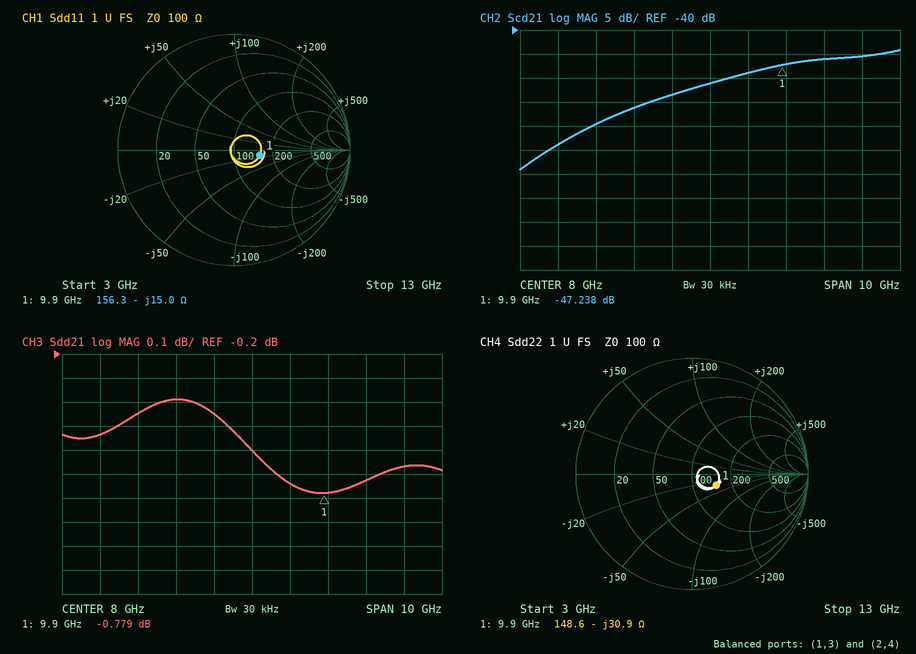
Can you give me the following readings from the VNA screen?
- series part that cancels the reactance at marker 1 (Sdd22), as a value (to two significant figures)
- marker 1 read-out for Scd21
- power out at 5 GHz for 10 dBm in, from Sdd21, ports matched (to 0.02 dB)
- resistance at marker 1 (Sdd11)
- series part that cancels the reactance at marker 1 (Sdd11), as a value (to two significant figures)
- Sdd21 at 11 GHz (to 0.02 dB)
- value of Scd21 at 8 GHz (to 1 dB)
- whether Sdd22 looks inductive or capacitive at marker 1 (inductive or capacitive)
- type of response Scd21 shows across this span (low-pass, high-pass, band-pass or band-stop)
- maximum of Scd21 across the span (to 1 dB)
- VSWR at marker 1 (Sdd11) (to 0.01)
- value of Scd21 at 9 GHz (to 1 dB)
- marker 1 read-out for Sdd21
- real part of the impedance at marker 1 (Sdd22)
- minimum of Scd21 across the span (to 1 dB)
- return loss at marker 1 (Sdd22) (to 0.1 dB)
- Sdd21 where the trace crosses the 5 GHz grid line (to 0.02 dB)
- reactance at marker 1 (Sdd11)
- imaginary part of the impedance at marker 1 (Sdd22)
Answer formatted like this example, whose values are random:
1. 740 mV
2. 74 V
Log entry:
1. 500 pH
2. -47.238 dB
3. 9.56 dBm
4. 156.3 Ω
5. 240 pH
6. -0.72 dB
7. -51 dB
8. capacitive
9. high-pass
10. -44 dB
11. 1.59
12. -49 dB
13. -0.779 dB
14. 148.6 Ω
15. -69 dB
16. 12.8 dB
17. -0.44 dB
18. -15.0 Ω
19. -30.9 Ω
